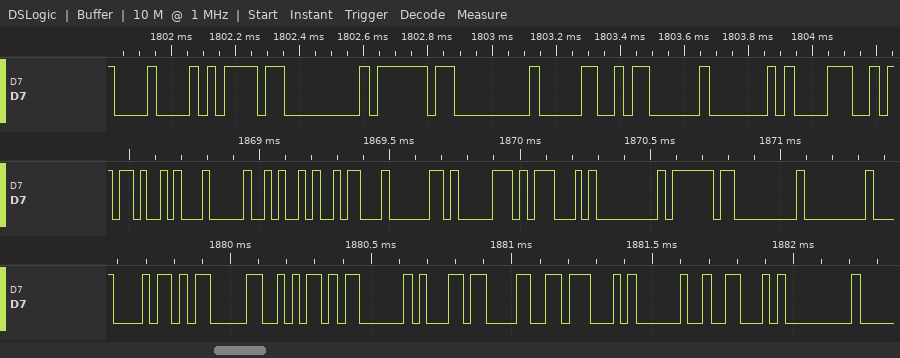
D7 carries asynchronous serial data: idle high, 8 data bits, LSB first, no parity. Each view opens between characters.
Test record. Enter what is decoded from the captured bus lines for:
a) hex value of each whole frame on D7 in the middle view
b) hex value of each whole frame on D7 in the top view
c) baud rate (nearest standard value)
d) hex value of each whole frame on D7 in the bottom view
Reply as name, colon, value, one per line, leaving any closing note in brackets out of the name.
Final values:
hex value of each whole frame on D7 in the middle view: 4B, 04, 4A, 1A, 60, 70, 47, 00, BF, 00, 00
hex value of each whole frame on D7 in the top view: 08, BD, 00, BF, 00, 30, 03, 40, 38
baud rate: 38400 baud
hex value of each whole frame on D7 in the bottom view: 68, 83, 6A, 03, B1, 98, 47, 20, 46, 00
